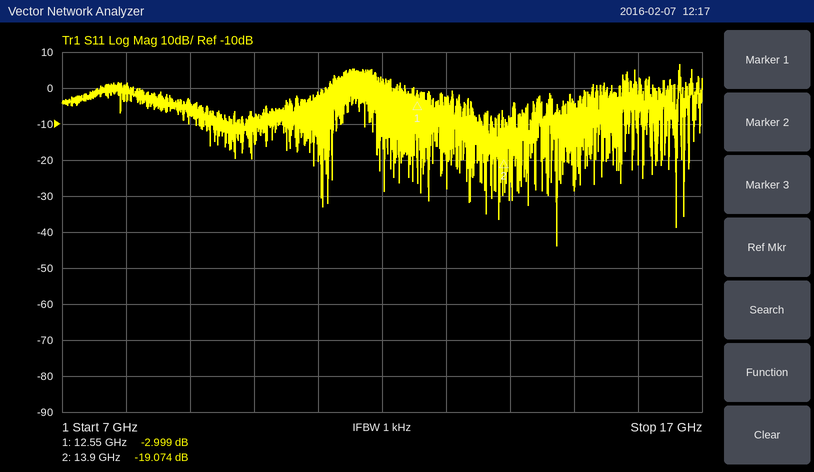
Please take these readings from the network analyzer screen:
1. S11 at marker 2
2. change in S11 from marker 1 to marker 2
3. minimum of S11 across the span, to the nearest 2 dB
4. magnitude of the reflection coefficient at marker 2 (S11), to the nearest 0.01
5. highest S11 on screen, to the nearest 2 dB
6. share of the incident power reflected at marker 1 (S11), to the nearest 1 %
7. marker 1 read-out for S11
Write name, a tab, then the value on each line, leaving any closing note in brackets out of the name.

S11 at marker 2	-19.074 dB
change in S11 from marker 1 to marker 2	-16.075 dB
minimum of S11 across the span, to the nearest 2 dB	-44 dB
magnitude of the reflection coefficient at marker 2 (S11), to the nearest 0.01	0.11
highest S11 on screen, to the nearest 2 dB	6 dB
share of the incident power reflected at marker 1 (S11), to the nearest 1 %	50 %
marker 1 read-out for S11	-2.999 dB
